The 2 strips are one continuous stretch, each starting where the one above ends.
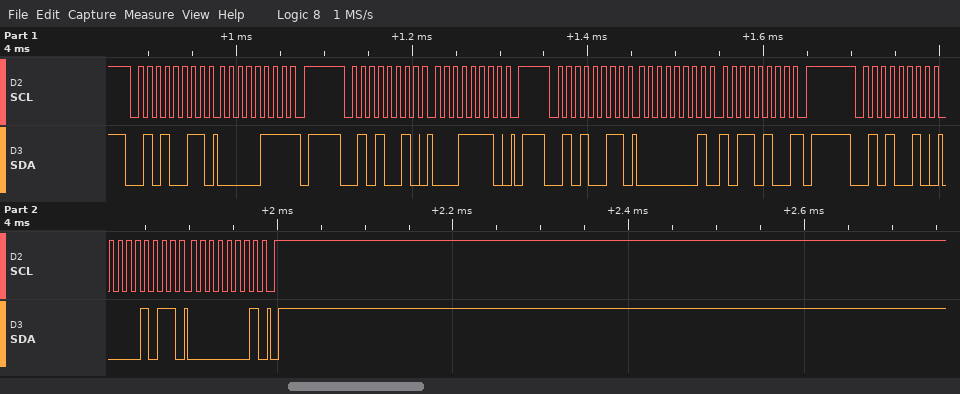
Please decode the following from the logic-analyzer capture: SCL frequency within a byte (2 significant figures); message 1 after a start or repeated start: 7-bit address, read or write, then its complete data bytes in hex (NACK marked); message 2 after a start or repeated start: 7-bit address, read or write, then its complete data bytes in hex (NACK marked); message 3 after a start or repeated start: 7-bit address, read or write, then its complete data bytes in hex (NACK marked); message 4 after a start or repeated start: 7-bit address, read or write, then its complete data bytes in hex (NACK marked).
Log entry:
100 kHz
0x29 read: 07 NACK
0x29 write: 1E
0x29 read: 01 B4 NACK
0x29 write: 0B 01
